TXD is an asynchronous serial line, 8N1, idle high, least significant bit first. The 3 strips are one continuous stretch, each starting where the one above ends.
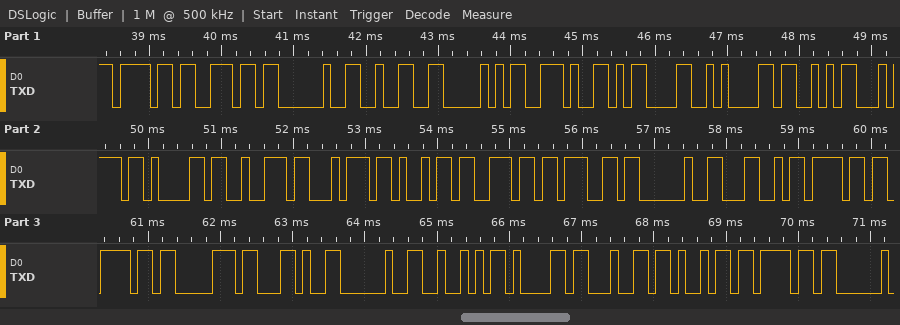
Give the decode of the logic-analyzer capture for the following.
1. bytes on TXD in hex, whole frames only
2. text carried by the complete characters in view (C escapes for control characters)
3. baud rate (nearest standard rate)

6F 6E 20 32 50 2E 0D 0A 53 74 61 72 74 69 6E 67 20 4C 6F 6F 70 2C 20 52 61 64 69 6F
"on 2P.\r\nStarting Loop, Radio"
9600 baud
